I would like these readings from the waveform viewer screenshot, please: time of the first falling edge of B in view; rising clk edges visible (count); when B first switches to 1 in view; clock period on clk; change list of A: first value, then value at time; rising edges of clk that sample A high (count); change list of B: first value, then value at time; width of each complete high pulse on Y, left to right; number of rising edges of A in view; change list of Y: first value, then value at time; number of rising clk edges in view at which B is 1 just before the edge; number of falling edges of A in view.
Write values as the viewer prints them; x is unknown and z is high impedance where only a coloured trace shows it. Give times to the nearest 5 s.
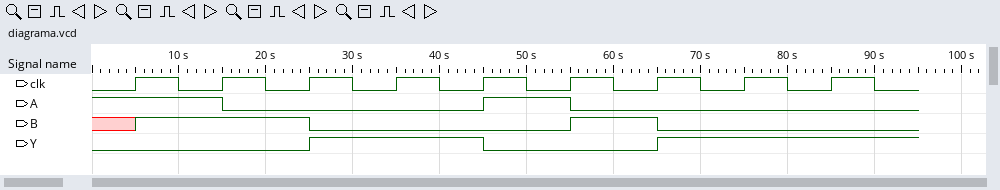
25 s
9
5 s
10 s
1, 0 at 15 s, 1 at 45 s, 0 at 55 s
3
x, 1 at 5 s, 0 at 25 s, 1 at 55 s, 0 at 65 s
20 s
1
0, 1 at 25 s, 0 at 45 s, 1 at 65 s
3
2
